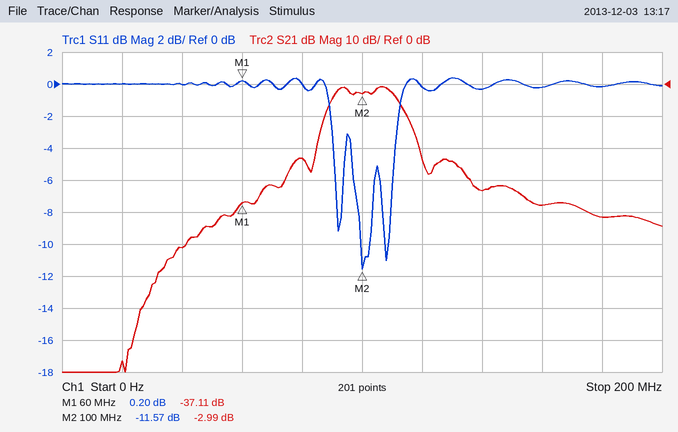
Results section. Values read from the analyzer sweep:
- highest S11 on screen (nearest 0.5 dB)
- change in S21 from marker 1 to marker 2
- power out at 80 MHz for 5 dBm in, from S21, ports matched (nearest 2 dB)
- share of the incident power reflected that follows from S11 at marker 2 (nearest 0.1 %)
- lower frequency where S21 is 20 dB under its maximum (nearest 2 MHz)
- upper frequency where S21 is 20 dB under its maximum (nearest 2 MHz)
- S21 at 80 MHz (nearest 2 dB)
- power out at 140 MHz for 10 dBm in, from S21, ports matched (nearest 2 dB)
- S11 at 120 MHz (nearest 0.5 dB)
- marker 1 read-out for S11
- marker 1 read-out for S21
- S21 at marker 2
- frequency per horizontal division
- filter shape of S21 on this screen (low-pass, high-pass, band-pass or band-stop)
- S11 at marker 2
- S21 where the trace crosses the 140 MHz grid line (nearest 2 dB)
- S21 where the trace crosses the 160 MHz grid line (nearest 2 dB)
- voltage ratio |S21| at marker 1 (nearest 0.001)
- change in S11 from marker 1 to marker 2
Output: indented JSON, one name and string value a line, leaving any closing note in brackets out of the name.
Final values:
{
  "highest S11 on screen": "0.5 dB",
  "change in S21 from marker 1 to marker 2": "34.12 dB",
  "power out at 80 MHz for 5 dBm in, from S21, ports matched": "-18 dBm",
  "share of the incident power reflected that follows from S11 at marker 2": "7.0 %",
  "lower frequency where S21 is 20 dB under its maximum": "84 MHz",
  "upper frequency where S21 is 20 dB under its maximum": "120 MHz",
  "S21 at 80 MHz": "-24 dB",
  "power out at 140 MHz for 10 dBm in, from S21, ports matched": "-24 dBm",
  "S11 at 120 MHz": "0.0 dB",
  "marker 1 read-out for S11": "0.20 dB",
  "marker 1 read-out for S21": "-37.11 dB",
  "S21 at marker 2": "-2.99 dB",
  "frequency per horizontal division": "20 MHz",
  "filter shape of S21 on this screen": "band-pass",
  "S11 at marker 2": "-11.57 dB",
  "S21 where the trace crosses the 140 MHz grid line": "-34 dB",
  "S21 where the trace crosses the 160 MHz grid line": "-38 dB",
  "voltage ratio |S21| at marker 1": "0.014",
  "change in S11 from marker 1 to marker 2": "-11.77 dB"
}
